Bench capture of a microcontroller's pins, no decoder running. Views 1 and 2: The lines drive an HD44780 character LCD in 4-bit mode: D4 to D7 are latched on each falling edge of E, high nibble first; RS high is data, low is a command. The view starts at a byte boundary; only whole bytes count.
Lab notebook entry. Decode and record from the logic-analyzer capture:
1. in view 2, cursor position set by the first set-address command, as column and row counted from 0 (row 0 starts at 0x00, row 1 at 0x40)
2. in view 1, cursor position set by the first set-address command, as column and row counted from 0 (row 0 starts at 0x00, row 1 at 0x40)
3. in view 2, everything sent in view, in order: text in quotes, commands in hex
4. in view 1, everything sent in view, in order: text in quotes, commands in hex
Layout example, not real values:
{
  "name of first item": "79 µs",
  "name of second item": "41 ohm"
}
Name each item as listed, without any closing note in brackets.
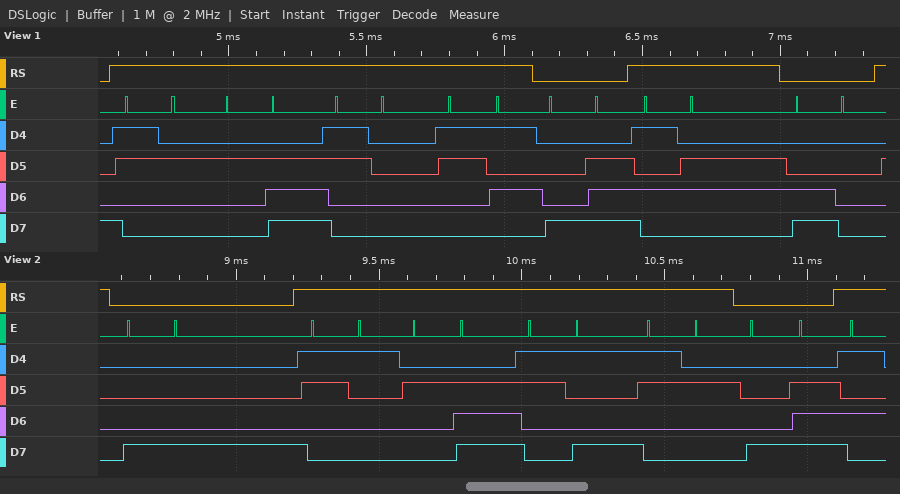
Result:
{
  "in view 2, cursor position set by the first set-address command, as column and row counted from 0": "column 8, row 0",
  "in view 1, cursor position set by the first set-address command, as column and row counted from 0": "column 14, row 0",
  "in view 2, everything sent in view, in order: text in quotes, commands in hex": "0x88 \"1.92\" 0x8E",
  "in view 1, everything sent in view, in order: text in quotes, commands in hex": "\"2.05\" 0x8E \"V\" 0xC0"
}
